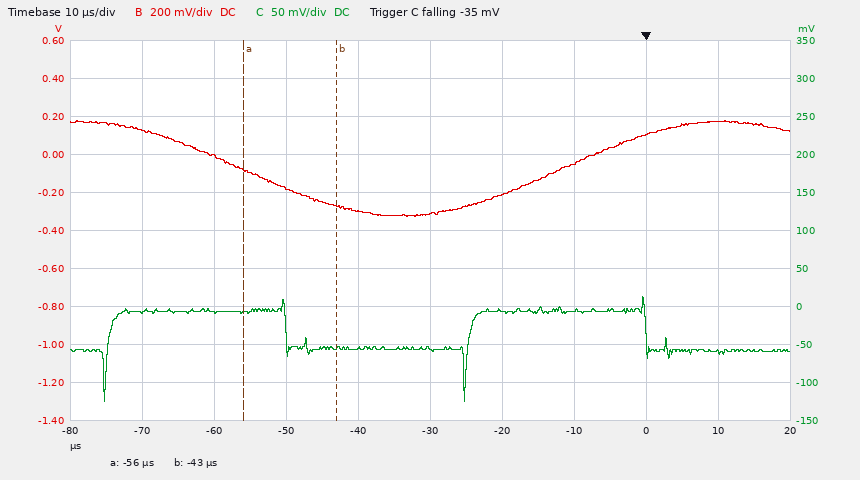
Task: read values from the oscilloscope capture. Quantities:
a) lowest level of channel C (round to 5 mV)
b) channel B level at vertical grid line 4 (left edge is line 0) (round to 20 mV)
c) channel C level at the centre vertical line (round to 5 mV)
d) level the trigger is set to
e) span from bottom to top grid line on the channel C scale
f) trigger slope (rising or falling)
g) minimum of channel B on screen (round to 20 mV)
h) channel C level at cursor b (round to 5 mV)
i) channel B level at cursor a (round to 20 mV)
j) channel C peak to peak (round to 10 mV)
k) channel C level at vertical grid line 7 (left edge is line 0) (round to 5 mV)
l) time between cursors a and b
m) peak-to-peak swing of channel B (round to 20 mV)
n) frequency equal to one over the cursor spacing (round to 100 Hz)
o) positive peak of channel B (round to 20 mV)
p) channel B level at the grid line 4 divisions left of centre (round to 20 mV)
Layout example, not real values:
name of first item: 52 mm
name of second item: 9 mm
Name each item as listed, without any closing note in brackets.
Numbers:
lowest level of channel C: -125 mV
channel B level at vertical grid line 4 (left edge is line 0): -300 mV
channel C level at the centre vertical line: -55 mV
level the trigger is set to: -35 mV
span from bottom to top grid line on the channel C scale: 500 mV
trigger slope: falling
minimum of channel B on screen: -320 mV
channel C level at cursor b: -55 mV
channel B level at cursor a: -80 mV
channel C peak to peak: 140 mV
channel C level at vertical grid line 7 (left edge is line 0): -5 mV
time between cursors a and b: 13 µs
peak-to-peak swing of channel B: 500 mV
frequency equal to one over the cursor spacing: 76.9 kHz
positive peak of channel B: 180 mV
channel B level at the grid line 4 divisions left of centre: 120 mV
